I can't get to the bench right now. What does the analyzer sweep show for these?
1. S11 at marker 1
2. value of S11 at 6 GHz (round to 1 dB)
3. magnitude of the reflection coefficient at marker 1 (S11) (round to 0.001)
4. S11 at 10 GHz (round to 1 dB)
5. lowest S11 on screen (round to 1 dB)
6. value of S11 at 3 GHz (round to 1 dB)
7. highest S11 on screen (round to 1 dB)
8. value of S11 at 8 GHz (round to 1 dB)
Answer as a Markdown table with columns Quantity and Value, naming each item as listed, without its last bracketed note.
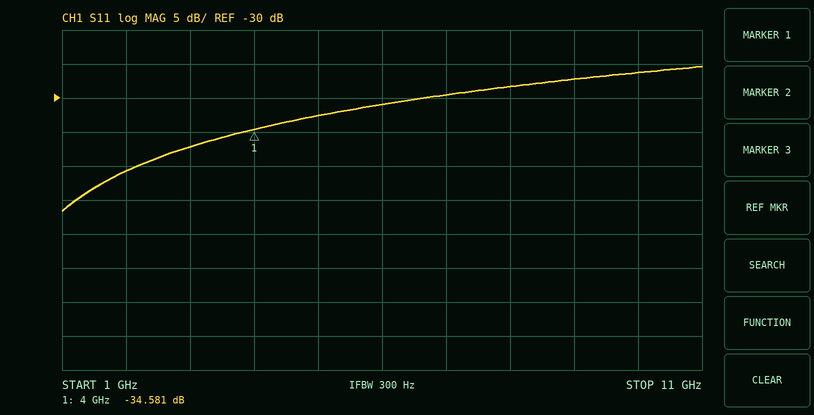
| Quantity | Value |
|---|---|
| S11 at marker 1 | -34.581 dB |
| value of S11 at 6 GHz | -31 dB |
| magnitude of the reflection coefficient at marker 1 (S11) | 0.019 |
| S11 at 10 GHz | -26 dB |
| lowest S11 on screen | -47 dB |
| value of S11 at 3 GHz | -37 dB |
| highest S11 on screen | -25 dB |
| value of S11 at 8 GHz | -28 dB |
